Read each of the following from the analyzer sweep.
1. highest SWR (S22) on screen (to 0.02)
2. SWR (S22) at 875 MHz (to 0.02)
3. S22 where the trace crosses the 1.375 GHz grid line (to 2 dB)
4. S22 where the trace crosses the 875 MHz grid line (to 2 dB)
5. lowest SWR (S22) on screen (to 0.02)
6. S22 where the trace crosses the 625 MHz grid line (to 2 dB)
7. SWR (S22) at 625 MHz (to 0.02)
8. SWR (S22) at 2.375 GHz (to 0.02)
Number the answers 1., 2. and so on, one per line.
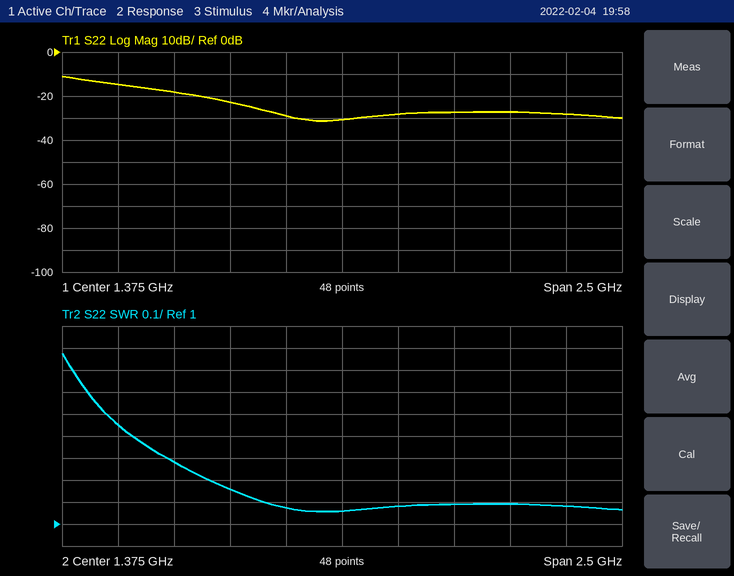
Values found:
1. 1.78
2. 1.16
3. -30 dB
4. -22 dB
5. 1.06
6. -18 dB
7. 1.28
8. 1.08
